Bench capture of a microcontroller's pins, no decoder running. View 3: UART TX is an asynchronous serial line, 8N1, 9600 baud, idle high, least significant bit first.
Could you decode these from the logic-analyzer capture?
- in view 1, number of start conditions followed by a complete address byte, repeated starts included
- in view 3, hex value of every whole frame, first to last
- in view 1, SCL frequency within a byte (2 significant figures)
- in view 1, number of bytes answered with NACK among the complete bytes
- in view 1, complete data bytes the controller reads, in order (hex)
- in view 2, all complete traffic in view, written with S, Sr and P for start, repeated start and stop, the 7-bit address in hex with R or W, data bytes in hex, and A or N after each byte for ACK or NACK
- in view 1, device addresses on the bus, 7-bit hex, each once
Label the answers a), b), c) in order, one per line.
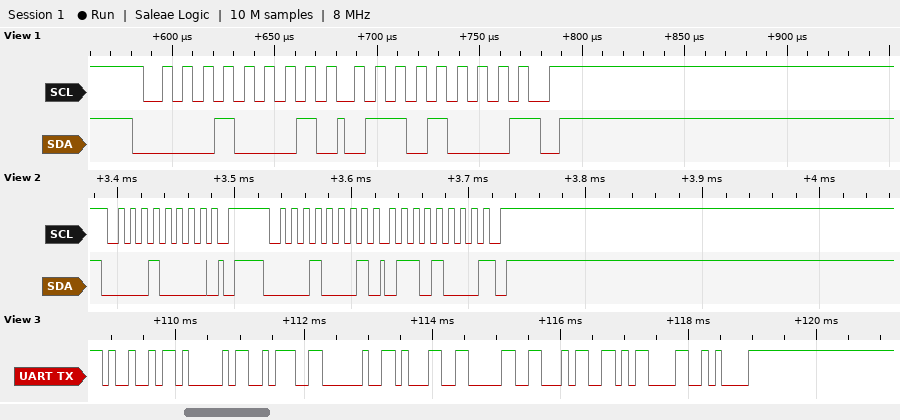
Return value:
a) 1
b) 49 41 3A 20 31 30 34 0D 0A
c) 100 kHz
d) 1
e) 68
f) S 08W A P S 08R A 68 N P
g) 0x08
